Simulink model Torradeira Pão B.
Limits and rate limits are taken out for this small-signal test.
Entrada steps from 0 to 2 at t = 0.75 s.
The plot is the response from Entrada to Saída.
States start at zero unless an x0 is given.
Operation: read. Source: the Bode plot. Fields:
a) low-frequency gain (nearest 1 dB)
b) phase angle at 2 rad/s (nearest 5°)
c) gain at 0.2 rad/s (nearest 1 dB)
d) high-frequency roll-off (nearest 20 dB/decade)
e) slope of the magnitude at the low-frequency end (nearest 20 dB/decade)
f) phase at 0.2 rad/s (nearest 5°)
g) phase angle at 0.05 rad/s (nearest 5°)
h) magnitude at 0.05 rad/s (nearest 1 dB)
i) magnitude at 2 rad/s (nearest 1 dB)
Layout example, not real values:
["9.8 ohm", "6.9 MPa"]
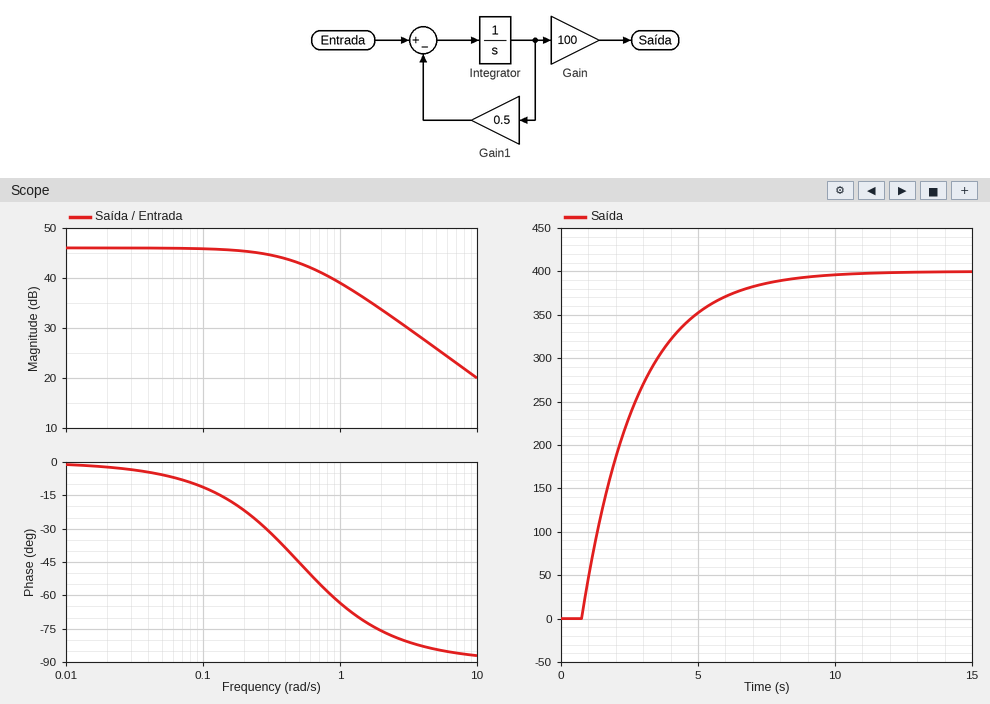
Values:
["46 dB", "-75°", "45 dB", "-20 dB/decade", "0 dB/decade", "-20°", "-5°", "46 dB", "34 dB"]
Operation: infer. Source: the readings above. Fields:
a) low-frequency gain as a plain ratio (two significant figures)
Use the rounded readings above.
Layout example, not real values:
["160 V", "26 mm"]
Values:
["200"]
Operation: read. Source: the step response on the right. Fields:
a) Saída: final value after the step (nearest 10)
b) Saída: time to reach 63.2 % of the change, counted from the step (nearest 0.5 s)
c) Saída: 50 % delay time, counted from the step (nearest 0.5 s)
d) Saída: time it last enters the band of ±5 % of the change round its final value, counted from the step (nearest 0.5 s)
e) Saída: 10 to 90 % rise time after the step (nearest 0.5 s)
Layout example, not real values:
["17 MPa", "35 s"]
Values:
["400", "2.0 s", "1.5 s", "6.0 s", "4.5 s"]
